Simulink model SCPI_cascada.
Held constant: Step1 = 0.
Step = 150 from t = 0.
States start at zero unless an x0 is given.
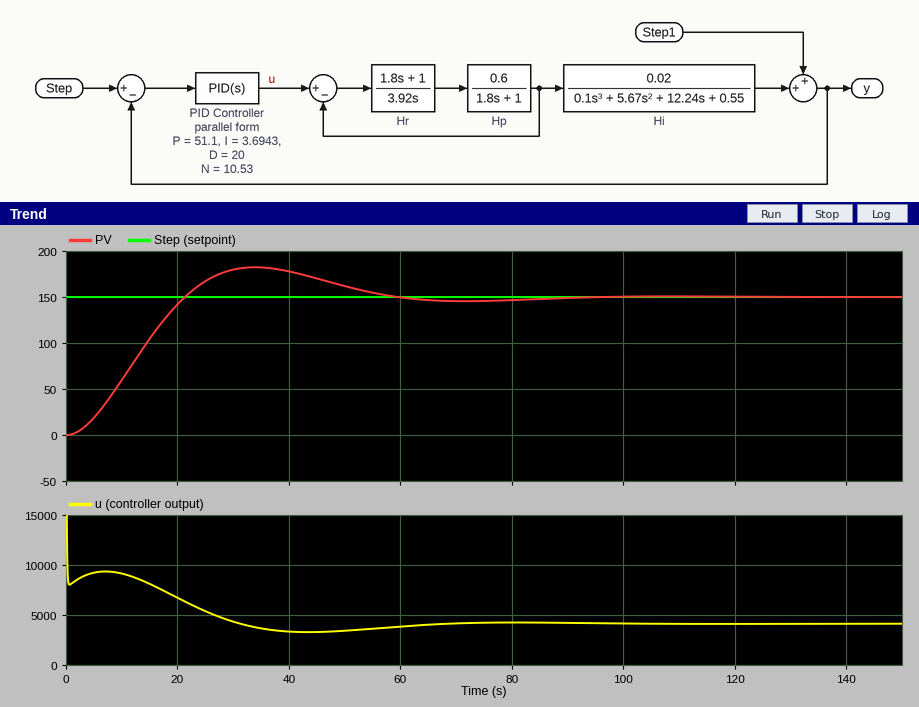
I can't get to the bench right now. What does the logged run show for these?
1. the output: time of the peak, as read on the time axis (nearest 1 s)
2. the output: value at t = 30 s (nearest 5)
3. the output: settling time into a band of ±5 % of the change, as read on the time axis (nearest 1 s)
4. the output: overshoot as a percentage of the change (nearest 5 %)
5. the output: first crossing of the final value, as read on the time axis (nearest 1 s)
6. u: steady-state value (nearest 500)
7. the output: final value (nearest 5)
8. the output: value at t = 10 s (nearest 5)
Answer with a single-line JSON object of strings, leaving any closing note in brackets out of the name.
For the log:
{"the output: time of the peak, as read on the time axis": "34 s", "the output: value at t = 30 s": "180", "the output: settling time into a band of ±5 % of the change, as read on the time axis": "53 s", "the output: overshoot as a percentage of the change": "20 %", "the output: first crossing of the final value, as read on the time axis": "21 s", "u: steady-state value": "4000", "the output: final value": "150", "the output: value at t = 10 s": "60"}
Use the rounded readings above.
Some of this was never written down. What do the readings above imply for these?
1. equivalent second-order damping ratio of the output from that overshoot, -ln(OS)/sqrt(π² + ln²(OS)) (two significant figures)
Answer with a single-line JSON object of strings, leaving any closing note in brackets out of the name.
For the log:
{"equivalent second-order damping ratio of the output from that overshoot, -ln(OS)/sqrt(π² + ln²(OS))": "0.46"}
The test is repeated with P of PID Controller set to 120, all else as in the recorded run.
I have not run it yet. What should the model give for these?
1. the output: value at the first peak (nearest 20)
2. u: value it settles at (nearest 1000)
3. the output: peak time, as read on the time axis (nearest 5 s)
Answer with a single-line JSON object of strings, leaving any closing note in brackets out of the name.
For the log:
{"the output: value at the first peak": "180", "u: value it settles at": "4000", "the output: peak time, as read on the time axis": "20 s"}
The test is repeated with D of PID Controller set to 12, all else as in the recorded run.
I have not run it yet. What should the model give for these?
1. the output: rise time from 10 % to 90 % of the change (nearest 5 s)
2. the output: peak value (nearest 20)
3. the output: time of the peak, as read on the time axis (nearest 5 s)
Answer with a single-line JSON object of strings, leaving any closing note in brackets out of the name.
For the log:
{"the output: rise time from 10 % to 90 % of the change": "15 s", "the output: peak value": "180", "the output: time of the peak, as read on the time axis": "35 s"}
